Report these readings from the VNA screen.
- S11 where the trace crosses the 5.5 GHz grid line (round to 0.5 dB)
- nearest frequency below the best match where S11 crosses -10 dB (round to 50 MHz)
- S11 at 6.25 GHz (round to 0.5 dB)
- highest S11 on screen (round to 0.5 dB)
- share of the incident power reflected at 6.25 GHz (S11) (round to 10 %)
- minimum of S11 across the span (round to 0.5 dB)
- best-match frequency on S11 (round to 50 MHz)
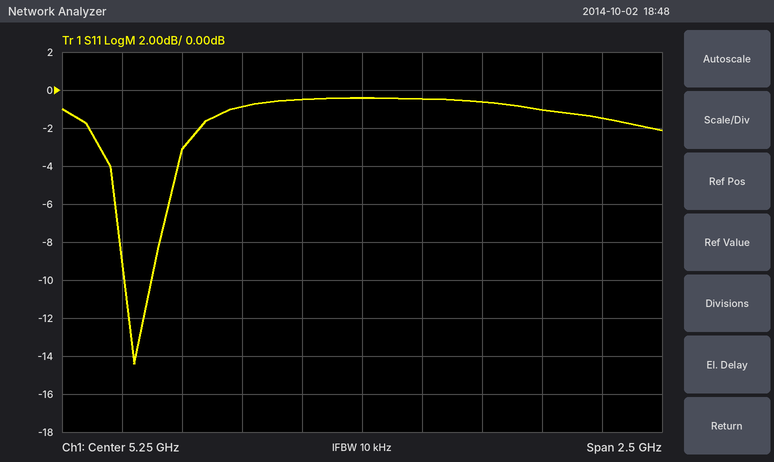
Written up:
-0.5 dB
4.25 GHz
-1.5 dB
-0.5 dB
70 %
-14.5 dB
4.30 GHz
